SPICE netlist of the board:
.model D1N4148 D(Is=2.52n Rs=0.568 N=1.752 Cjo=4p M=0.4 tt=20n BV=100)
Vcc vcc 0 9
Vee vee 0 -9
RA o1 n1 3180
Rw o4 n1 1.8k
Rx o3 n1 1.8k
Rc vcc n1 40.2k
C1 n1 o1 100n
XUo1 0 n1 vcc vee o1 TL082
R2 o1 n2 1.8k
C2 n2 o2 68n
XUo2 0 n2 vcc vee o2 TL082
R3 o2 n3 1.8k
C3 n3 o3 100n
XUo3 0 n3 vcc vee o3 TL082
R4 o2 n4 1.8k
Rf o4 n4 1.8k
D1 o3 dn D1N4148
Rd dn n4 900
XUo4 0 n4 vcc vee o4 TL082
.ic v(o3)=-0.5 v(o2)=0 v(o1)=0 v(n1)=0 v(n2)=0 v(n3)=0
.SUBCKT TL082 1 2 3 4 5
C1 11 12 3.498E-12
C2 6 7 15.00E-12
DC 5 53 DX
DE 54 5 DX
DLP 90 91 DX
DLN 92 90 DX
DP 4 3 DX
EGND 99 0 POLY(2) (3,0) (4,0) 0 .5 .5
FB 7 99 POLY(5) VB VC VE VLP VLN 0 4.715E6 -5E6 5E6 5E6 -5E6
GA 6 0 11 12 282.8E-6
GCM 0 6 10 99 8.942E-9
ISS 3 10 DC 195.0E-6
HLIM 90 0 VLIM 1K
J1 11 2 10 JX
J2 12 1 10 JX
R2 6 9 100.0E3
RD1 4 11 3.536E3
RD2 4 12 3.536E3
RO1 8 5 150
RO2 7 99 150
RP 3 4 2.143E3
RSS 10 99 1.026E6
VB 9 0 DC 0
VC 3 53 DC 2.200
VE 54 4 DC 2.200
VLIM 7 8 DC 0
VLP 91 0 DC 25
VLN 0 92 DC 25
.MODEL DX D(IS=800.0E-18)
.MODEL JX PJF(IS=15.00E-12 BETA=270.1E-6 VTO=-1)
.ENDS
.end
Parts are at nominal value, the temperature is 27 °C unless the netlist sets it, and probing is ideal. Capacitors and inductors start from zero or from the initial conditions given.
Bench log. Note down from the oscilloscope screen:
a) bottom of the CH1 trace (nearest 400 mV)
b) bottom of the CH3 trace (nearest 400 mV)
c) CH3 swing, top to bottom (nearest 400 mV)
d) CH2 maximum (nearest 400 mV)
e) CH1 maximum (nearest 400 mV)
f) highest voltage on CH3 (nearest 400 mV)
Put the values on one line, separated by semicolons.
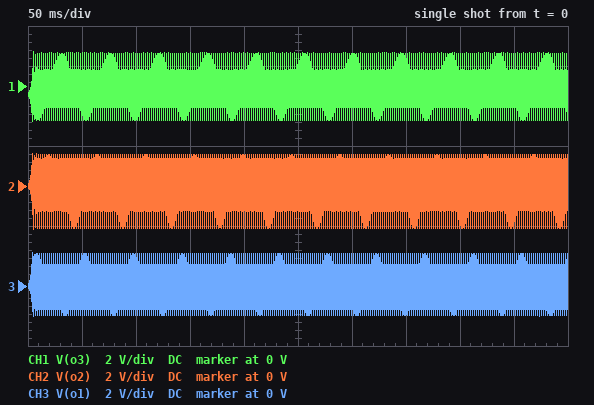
-1.6 V; -1.6 V; 3.2 V; 1.6 V; 1.6 V; 1.6 V
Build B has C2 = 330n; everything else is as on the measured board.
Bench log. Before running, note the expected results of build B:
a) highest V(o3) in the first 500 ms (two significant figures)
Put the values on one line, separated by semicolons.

7.5 V
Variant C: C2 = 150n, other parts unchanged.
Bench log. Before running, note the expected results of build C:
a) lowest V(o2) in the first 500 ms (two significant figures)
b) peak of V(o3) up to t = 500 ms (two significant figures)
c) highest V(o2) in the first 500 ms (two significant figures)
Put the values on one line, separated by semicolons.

-1.5 V; 1.8 V; 1.0 V
